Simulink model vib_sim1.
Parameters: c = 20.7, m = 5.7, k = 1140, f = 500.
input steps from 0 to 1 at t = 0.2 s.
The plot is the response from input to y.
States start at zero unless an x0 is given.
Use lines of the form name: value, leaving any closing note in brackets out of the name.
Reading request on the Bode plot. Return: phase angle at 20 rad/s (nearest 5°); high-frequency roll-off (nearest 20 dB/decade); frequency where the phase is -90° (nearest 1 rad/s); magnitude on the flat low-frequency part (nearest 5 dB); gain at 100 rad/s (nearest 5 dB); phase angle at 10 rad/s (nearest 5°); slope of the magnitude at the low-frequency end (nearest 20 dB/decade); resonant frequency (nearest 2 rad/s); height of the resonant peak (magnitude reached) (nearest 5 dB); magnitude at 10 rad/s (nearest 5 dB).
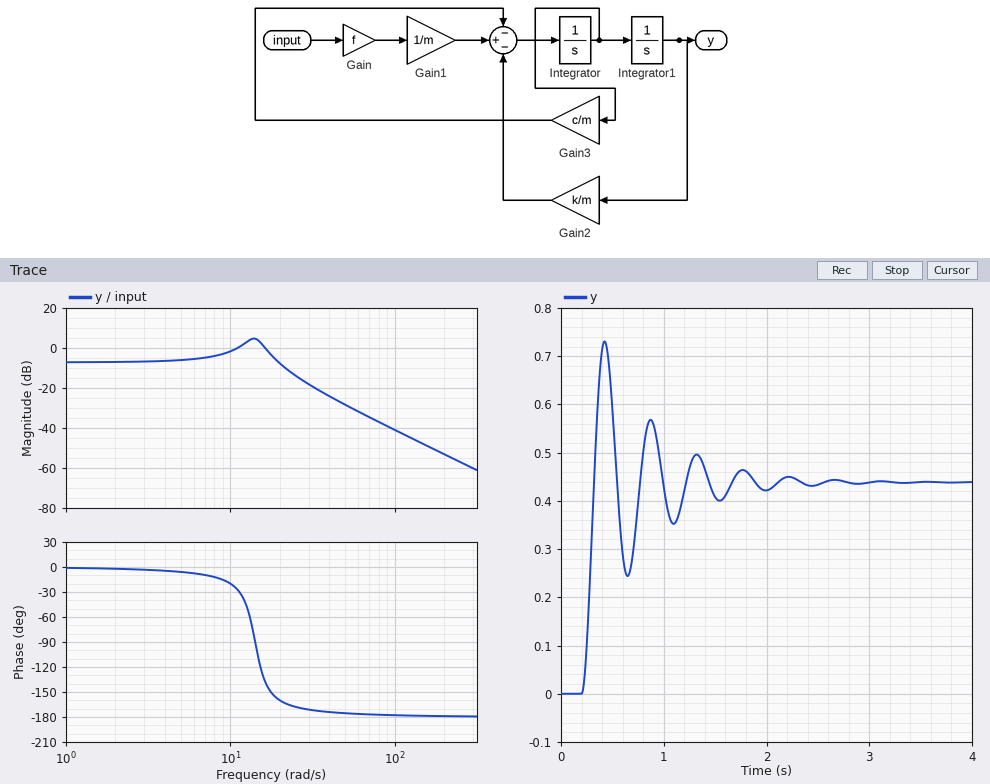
phase angle at 20 rad/s: -160°
high-frequency roll-off: -40 dB/decade
frequency where the phase is -90°: 14 rad/s
magnitude on the flat low-frequency part: -5 dB
gain at 100 rad/s: -40 dB
phase angle at 10 rad/s: -20°
slope of the magnitude at the low-frequency end: 0 dB/decade
resonant frequency: 14 rad/s
height of the resonant peak (magnitude reached): 5 dB
magnitude at 10 rad/s: 0 dB
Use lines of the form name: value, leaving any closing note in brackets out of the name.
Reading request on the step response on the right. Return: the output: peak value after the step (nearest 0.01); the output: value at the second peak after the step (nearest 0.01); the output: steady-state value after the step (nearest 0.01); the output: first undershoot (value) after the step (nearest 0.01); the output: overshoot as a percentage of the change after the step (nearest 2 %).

the output: peak value after the step: 0.73
the output: value at the second peak after the step: 0.57
the output: steady-state value after the step: 0.44
the output: first undershoot (value) after the step: 0.24
the output: overshoot as a percentage of the change after the step: 66 %
